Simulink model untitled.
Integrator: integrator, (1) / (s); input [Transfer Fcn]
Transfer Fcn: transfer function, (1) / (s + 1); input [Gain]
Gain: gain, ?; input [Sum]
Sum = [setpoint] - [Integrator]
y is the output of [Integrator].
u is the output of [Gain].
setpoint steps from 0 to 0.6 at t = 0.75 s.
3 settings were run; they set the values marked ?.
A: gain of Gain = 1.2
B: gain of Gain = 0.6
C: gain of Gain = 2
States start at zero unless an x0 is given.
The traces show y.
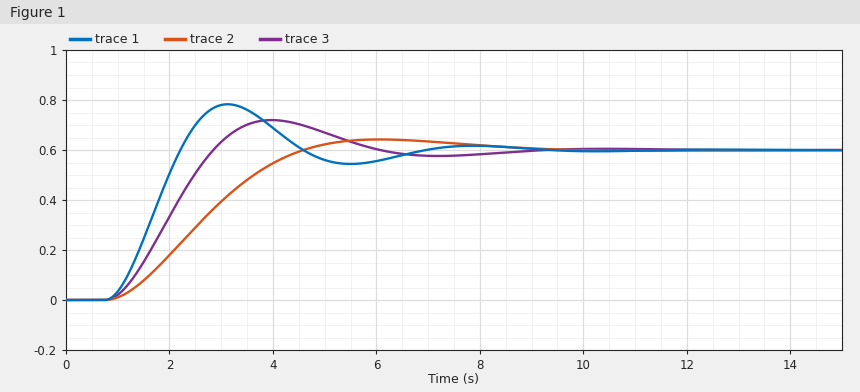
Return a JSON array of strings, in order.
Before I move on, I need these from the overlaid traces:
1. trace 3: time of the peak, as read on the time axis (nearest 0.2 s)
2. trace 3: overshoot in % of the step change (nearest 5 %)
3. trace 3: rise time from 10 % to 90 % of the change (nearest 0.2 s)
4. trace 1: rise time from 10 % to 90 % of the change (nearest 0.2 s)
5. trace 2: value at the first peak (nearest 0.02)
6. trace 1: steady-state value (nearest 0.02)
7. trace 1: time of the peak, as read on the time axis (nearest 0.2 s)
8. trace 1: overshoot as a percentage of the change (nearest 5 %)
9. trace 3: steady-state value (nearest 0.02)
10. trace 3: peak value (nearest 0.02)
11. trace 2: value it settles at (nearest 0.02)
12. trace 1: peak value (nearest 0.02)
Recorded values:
["4.0 s", "20 %", "1.4 s", "1.0 s", "0.64", "0.60", "3.2 s", "30 %", "0.60", "0.72", "0.60", "0.78"]
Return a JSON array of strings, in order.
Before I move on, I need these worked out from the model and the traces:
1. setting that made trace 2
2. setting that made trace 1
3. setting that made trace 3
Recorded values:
["B", "C", "A"]
